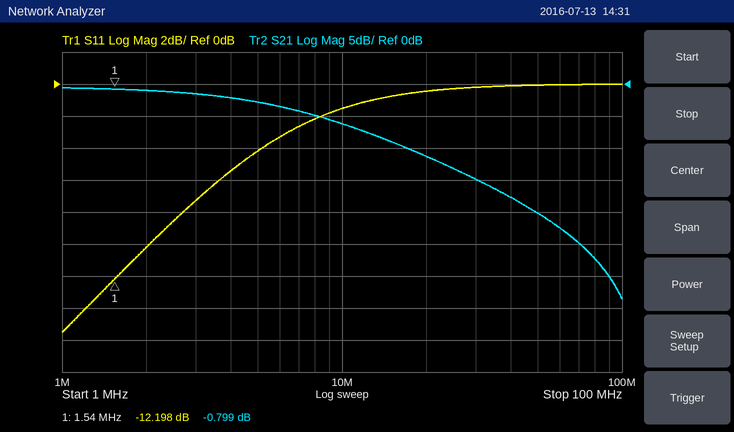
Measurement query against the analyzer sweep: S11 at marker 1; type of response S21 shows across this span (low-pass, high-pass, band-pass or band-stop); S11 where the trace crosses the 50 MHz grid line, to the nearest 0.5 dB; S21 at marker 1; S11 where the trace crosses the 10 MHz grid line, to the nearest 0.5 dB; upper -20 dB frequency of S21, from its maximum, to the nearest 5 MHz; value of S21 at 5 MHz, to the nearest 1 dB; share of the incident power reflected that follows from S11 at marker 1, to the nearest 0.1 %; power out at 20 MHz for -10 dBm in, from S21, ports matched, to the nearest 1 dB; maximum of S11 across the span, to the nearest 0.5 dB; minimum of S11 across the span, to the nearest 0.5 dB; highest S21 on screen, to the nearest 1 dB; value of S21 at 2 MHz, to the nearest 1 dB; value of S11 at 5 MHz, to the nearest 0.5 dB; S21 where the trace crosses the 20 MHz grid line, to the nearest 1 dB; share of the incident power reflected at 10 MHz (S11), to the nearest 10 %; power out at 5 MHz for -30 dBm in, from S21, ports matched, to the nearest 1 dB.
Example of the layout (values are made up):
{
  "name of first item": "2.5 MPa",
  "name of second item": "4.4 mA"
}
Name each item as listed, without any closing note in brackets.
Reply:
{
  "S11 at marker 1": "-12.198 dB",
  "type of response S21 shows across this span": "low-pass",
  "S11 where the trace crosses the 50 MHz grid line, to the nearest 0.5 dB": "0.0 dB",
  "S21 at marker 1": "-0.799 dB",
  "S11 where the trace crosses the 10 MHz grid line, to the nearest 0.5 dB": "-1.5 dB",
  "upper -20 dB frequency of S21, from its maximum, to the nearest 5 MHz": "50 MHz",
  "value of S21 at 5 MHz, to the nearest 1 dB": "-3 dB",
  "share of the incident power reflected that follows from S11 at marker 1, to the nearest 0.1 %": "6.0 %",
  "power out at 20 MHz for -10 dBm in, from S21, ports matched, to the nearest 1 dB": "-21 dBm",
  "maximum of S11 across the span, to the nearest 0.5 dB": "0.0 dB",
  "minimum of S11 across the span, to the nearest 0.5 dB": "-15.5 dB",
  "highest S21 on screen, to the nearest 1 dB": "-1 dB",
  "value of S21 at 2 MHz, to the nearest 1 dB": "-1 dB",
  "value of S11 at 5 MHz, to the nearest 0.5 dB": "-4.0 dB",
  "S21 where the trace crosses the 20 MHz grid line, to the nearest 1 dB": "-11 dB",
  "share of the incident power reflected at 10 MHz (S11), to the nearest 10 %": "70 %",
  "power out at 5 MHz for -30 dBm in, from S21, ports matched, to the nearest 1 dB": "-33 dBm"
}
